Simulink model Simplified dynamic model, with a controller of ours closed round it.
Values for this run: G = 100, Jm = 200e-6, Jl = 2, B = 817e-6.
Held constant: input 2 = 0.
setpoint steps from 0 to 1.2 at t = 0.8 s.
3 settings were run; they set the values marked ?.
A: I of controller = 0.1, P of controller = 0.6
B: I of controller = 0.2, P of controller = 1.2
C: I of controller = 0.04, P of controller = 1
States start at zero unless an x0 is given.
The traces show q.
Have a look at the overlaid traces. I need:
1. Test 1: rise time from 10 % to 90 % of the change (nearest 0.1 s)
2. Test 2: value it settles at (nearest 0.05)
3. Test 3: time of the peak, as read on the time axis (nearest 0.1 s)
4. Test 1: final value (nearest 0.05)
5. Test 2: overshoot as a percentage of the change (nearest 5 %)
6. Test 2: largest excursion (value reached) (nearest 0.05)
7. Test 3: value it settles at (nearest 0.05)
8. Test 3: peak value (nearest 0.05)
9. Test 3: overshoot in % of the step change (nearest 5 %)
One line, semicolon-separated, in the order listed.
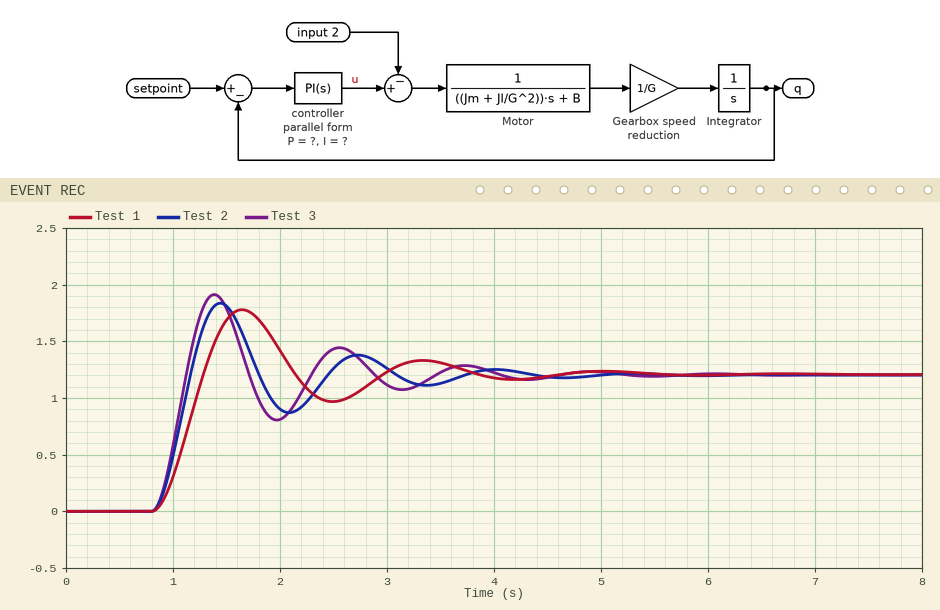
0.3 s; 1.20; 1.4 s; 1.20; 55 %; 1.85; 1.20; 1.90; 60 %
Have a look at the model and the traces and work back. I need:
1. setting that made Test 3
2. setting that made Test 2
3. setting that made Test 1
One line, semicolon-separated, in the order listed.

B; C; A
